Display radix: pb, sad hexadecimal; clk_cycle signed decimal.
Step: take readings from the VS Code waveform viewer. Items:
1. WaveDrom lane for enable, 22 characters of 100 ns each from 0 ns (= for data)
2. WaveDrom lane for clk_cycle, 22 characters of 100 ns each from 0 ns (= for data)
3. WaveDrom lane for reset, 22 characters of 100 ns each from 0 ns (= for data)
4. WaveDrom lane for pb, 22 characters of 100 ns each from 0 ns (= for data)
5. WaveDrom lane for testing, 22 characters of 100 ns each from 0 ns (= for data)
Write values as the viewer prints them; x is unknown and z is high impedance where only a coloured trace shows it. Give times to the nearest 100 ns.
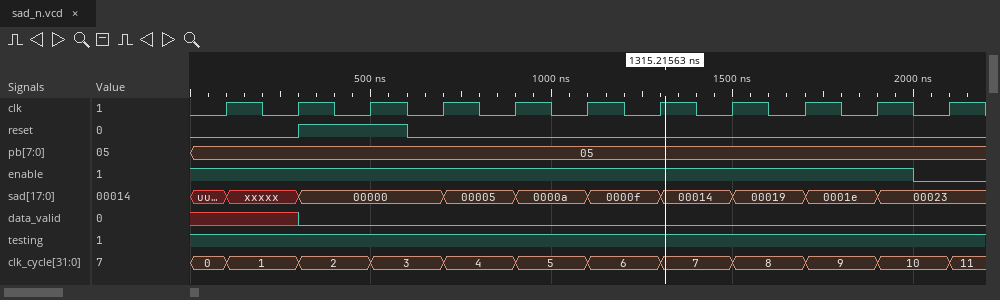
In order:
{name: 'enable', wave: '1...................0.'}
{name: 'clk_cycle', wave: '==.=.=.=.=.=.=.=.=.=.=', data: '0 1 2 3 4 5 6 7 8 9 10 11'}
{name: 'reset', wave: '0..1..0...............'}
{name: 'pb', wave: '=.....................', data: '05'}
{name: 'testing', wave: '1.....................'}
